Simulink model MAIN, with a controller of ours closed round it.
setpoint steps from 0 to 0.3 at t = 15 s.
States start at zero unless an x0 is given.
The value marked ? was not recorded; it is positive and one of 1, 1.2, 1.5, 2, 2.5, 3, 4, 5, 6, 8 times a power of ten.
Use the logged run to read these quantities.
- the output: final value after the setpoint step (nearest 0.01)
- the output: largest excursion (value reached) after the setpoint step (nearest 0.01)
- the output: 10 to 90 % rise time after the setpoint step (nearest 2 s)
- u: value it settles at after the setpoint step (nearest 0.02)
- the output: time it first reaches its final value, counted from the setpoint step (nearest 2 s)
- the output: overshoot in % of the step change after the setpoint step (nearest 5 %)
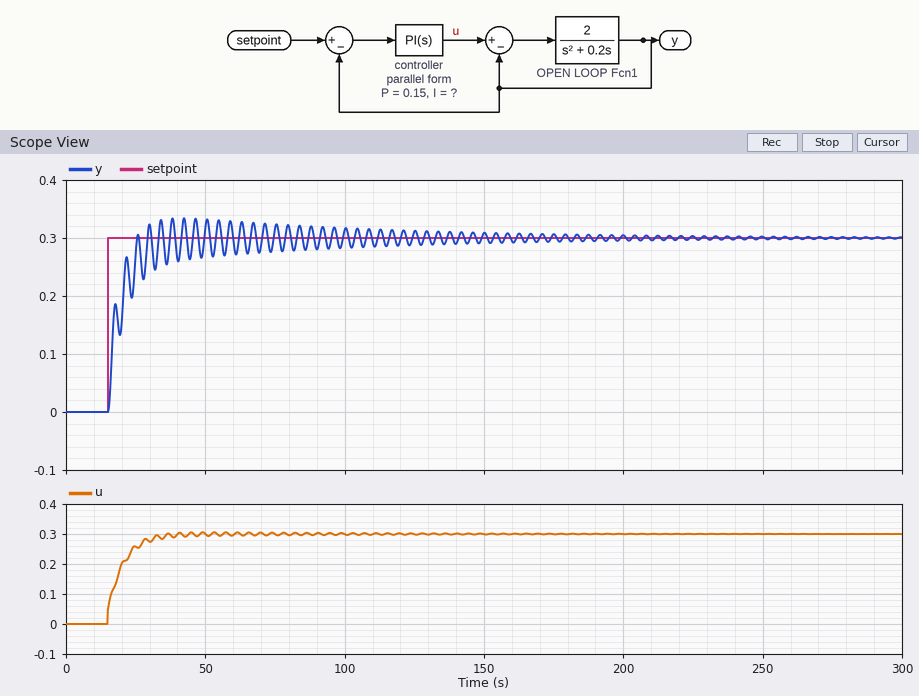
0.30
0.33
10 s
0.30
10 s
10 %
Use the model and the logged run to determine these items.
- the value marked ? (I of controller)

0.2
